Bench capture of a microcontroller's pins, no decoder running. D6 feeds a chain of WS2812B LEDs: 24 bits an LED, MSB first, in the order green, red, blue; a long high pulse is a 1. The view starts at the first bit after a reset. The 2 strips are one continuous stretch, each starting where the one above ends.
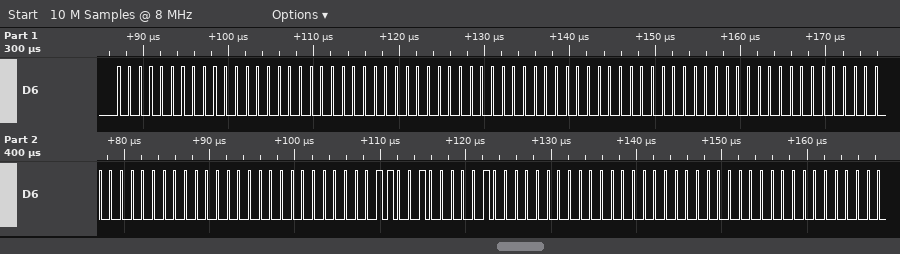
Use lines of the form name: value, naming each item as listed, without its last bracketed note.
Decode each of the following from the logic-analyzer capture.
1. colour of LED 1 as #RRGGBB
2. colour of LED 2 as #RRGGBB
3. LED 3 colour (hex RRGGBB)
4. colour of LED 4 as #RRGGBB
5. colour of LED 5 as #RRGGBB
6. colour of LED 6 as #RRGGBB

colour of LED 1 as #RRGGBB: #000000
colour of LED 2 as #RRGGBB: #000000
LED 3 colour: #000000
colour of LED 4 as #RRGGBB: #000000
colour of LED 5 as #RRGGBB: #083200
colour of LED 6 as #RRGGBB: #000000
